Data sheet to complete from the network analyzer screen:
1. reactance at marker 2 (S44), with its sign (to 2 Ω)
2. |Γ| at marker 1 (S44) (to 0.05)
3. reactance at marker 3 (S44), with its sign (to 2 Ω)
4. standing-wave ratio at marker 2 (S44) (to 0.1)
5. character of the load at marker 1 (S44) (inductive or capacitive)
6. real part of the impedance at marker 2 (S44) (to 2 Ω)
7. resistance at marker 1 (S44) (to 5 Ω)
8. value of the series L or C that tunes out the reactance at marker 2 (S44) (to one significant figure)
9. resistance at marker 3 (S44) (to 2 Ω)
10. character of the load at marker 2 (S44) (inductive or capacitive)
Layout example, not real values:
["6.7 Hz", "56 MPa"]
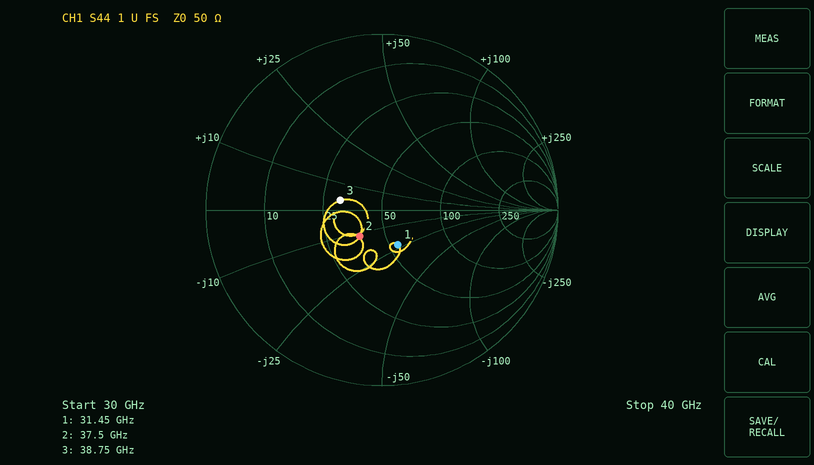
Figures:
["-12 Ω", "0.20", "+4 Ω", "1.5", "capacitive", "38 Ω", "55 Ω", "50 pH", "30 Ω", "capacitive"]
